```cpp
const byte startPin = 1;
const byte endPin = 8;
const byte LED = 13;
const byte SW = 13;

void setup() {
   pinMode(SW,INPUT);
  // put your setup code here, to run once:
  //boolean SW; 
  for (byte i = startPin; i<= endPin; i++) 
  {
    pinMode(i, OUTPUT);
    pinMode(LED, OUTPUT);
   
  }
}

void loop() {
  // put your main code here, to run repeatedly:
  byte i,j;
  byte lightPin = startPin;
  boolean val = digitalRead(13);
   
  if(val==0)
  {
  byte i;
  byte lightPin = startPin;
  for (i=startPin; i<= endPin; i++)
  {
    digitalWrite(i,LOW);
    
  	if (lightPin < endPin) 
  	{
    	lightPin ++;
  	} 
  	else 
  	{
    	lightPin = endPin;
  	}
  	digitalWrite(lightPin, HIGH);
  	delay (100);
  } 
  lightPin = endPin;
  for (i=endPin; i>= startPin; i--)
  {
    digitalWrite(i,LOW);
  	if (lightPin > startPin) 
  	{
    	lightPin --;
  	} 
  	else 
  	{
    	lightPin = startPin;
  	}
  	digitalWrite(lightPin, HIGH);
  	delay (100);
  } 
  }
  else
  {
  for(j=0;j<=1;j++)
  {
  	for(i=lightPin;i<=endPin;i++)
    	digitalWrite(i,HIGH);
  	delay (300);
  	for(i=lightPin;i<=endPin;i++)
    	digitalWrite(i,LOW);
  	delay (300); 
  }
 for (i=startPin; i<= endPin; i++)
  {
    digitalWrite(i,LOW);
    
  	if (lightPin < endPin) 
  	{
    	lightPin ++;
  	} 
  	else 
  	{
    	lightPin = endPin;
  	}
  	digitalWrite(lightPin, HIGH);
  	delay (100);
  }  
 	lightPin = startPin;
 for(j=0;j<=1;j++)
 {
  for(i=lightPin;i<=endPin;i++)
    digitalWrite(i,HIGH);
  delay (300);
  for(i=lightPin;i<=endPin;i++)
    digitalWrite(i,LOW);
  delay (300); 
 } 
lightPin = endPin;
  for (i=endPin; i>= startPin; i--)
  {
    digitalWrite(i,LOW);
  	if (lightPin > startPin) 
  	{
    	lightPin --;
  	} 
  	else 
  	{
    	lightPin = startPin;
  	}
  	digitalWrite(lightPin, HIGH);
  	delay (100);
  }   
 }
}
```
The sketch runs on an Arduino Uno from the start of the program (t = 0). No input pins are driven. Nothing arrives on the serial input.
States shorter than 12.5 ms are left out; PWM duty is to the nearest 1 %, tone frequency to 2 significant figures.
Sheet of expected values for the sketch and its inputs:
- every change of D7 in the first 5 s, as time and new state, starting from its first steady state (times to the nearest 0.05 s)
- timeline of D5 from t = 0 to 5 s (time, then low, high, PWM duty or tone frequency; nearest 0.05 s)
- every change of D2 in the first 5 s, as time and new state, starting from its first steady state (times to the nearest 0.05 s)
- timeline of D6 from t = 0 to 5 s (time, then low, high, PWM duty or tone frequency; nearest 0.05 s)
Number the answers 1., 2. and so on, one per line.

1. 0 s low; 0.5 s high; 0.6 s low; 0.8 s high; 0.9 s low; 2.1 s high; 2.2 s low; 2.4 s high; 2.5 s low; 3.7 s high; 3.8 s low; 4 s high; 4.1 s low
2. 0 s low; 0.3 s high; 0.4 s low; 1 s high; 1.1 s low; 1.9 s high; 2 s low; 2.6 s high; 2.7 s low; 3.5 s high; 3.6 s low; 4.2 s high; 4.3 s low
3. 0 s high; 0.1 s low; 1.3 s high; 1.4 s low; 1.6 s high; 1.7 s low; 2.9 s high; 3 s low; 3.2 s high; 3.3 s low; 4.5 s high; 4.6 s low; 4.8 s high; 4.9 s low
4. 0 s low; 0.4 s high; 0.5 s low; 0.9 s high; 1 s low; 2 s high; 2.1 s low; 2.5 s high; 2.6 s low; 3.6 s high; 3.7 s low; 4.1 s high; 4.2 s low
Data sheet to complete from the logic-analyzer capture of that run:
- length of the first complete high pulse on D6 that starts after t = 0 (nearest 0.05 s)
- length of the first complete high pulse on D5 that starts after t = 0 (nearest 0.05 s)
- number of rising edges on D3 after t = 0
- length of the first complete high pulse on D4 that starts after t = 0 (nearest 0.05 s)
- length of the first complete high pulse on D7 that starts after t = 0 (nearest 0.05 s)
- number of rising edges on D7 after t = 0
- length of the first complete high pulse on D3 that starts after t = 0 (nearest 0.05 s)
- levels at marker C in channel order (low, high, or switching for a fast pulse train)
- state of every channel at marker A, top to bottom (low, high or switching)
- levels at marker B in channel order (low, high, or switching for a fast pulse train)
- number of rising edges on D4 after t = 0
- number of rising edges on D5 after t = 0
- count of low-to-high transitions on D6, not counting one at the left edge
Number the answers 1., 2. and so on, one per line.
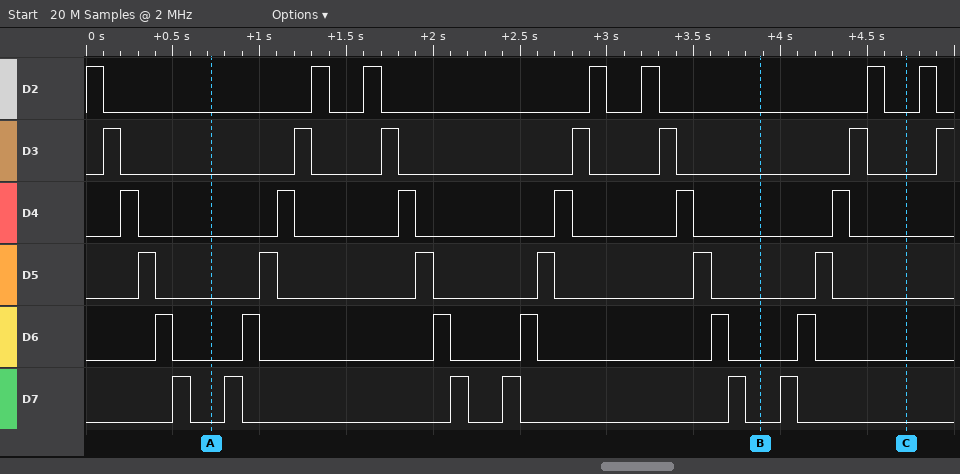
1. 0.10 s
2. 0.10 s
3. 7
4. 0.10 s
5. 0.10 s
6. 6
7. 0.10 s
8. D2 low, D3 low, D4 low, D5 low, D6 low, D7 low
9. D2 low, D3 low, D4 low, D5 low, D6 low, D7 low
10. D2 low, D3 low, D4 low, D5 low, D6 low, D7 low
11. 6
12. 6
13. 6
